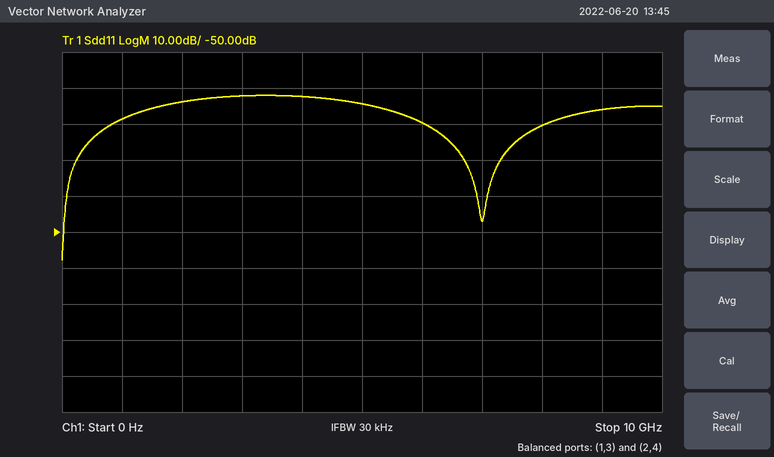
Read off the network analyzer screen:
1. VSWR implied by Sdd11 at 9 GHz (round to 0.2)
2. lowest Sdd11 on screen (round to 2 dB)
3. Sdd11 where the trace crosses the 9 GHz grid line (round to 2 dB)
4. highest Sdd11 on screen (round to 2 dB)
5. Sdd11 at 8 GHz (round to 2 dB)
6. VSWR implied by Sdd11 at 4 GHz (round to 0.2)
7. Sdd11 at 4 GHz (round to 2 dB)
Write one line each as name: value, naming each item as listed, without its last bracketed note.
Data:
VSWR implied by Sdd11 at 9 GHz: 1.4
lowest Sdd11 on screen: -58 dB
Sdd11 where the trace crosses the 9 GHz grid line: -16 dB
highest Sdd11 on screen: -12 dB
Sdd11 at 8 GHz: -20 dB
VSWR implied by Sdd11 at 4 GHz: 1.6
Sdd11 at 4 GHz: -12 dB
